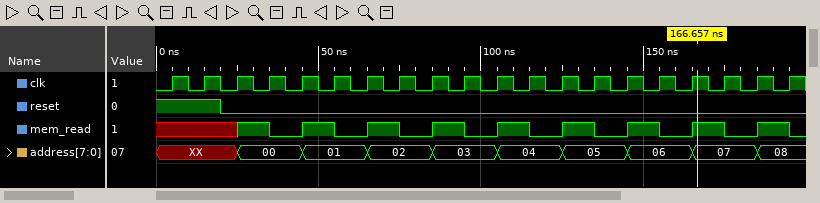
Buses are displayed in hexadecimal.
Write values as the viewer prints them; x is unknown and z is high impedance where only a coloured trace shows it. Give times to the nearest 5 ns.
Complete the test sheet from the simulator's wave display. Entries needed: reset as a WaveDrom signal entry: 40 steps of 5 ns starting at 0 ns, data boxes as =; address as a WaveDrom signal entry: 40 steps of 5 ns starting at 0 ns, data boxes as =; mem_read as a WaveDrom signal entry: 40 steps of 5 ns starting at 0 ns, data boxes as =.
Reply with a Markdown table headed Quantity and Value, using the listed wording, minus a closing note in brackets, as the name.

| Quantity | Value |
|---|---|
| reset as a WaveDrom signal entry: 40 steps of 5 ns starting at 0 ns, data boxes as = | {name: 'reset', wave: '1...0...................................'} |
| address as a WaveDrom signal entry: 40 steps of 5 ns starting at 0 ns, data boxes as = | {name: 'address', wave: 'x....=...=...=...=...=...=...=...=...=..', data: '00 01 02 03 04 05 06 07 08'} |
| mem_read as a WaveDrom signal entry: 40 steps of 5 ns starting at 0 ns, data boxes as = | {name: 'mem_read', wave: 'x....1.0.1.0.1.0.1.0.1.0.1.0.1.0.1.0.1.0'} |
